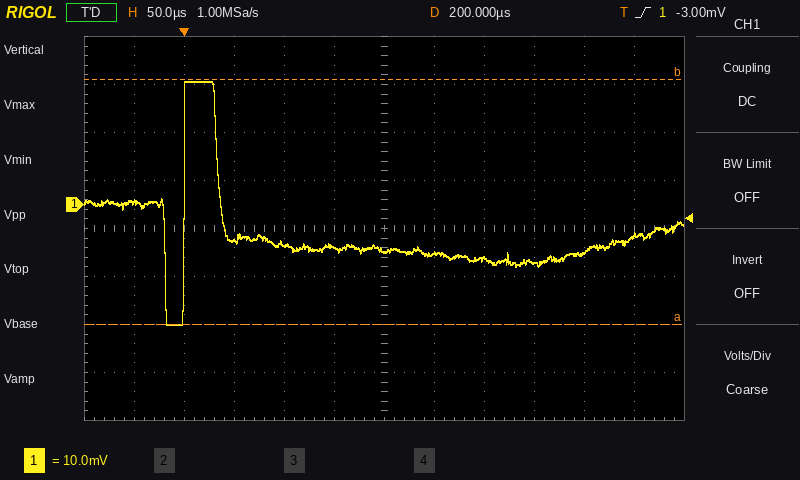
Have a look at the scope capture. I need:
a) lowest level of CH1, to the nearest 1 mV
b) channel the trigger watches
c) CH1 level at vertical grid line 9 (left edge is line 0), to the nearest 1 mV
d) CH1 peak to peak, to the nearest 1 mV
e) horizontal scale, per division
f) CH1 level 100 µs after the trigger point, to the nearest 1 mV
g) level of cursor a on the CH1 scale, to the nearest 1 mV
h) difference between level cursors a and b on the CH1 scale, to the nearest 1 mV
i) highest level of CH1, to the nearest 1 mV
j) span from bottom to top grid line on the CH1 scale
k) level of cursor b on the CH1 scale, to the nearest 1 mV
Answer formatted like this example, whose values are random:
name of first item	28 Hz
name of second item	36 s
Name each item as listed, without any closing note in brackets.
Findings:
lowest level of CH1, to the nearest 1 mV	-25 mV
channel the trigger watches	CH1
CH1 level at vertical grid line 9 (left edge is line 0), to the nearest 1 mV	-12 mV
CH1 peak to peak, to the nearest 1 mV	51 mV
horizontal scale, per division	50 µs
CH1 level 100 µs after the trigger point, to the nearest 1 mV	-8 mV
level of cursor a on the CH1 scale, to the nearest 1 mV	-25 mV
difference between level cursors a and b on the CH1 scale, to the nearest 1 mV	51 mV
highest level of CH1, to the nearest 1 mV	26 mV
span from bottom to top grid line on the CH1 scale	80 mV
level of cursor b on the CH1 scale, to the nearest 1 mV	26 mV
